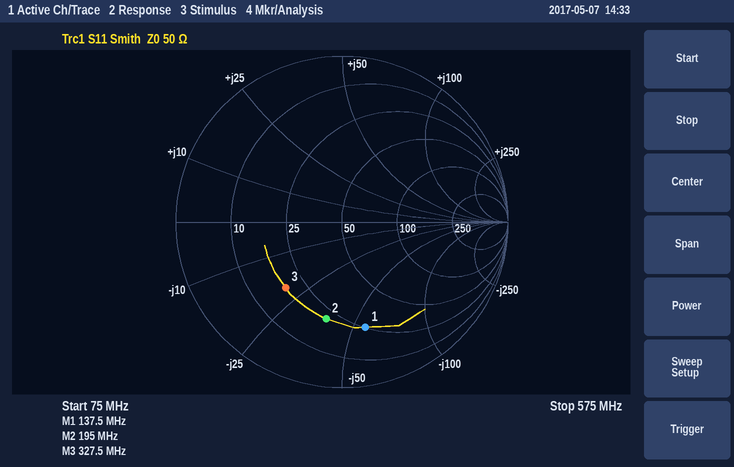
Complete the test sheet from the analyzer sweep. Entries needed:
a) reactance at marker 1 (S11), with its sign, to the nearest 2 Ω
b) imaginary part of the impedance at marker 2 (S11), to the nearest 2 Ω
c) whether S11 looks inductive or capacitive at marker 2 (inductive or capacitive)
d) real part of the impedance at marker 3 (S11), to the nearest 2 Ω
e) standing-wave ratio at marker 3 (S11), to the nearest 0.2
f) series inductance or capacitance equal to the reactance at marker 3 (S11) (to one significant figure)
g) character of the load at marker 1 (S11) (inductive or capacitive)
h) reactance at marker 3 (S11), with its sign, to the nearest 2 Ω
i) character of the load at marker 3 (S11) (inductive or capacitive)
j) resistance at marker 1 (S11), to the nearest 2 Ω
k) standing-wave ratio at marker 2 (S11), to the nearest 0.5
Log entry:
-56 Ω
-38 Ω
capacitive
18 Ω
3.2
20 pF
capacitive
-20 Ω
capacitive
26 Ω
4.0
